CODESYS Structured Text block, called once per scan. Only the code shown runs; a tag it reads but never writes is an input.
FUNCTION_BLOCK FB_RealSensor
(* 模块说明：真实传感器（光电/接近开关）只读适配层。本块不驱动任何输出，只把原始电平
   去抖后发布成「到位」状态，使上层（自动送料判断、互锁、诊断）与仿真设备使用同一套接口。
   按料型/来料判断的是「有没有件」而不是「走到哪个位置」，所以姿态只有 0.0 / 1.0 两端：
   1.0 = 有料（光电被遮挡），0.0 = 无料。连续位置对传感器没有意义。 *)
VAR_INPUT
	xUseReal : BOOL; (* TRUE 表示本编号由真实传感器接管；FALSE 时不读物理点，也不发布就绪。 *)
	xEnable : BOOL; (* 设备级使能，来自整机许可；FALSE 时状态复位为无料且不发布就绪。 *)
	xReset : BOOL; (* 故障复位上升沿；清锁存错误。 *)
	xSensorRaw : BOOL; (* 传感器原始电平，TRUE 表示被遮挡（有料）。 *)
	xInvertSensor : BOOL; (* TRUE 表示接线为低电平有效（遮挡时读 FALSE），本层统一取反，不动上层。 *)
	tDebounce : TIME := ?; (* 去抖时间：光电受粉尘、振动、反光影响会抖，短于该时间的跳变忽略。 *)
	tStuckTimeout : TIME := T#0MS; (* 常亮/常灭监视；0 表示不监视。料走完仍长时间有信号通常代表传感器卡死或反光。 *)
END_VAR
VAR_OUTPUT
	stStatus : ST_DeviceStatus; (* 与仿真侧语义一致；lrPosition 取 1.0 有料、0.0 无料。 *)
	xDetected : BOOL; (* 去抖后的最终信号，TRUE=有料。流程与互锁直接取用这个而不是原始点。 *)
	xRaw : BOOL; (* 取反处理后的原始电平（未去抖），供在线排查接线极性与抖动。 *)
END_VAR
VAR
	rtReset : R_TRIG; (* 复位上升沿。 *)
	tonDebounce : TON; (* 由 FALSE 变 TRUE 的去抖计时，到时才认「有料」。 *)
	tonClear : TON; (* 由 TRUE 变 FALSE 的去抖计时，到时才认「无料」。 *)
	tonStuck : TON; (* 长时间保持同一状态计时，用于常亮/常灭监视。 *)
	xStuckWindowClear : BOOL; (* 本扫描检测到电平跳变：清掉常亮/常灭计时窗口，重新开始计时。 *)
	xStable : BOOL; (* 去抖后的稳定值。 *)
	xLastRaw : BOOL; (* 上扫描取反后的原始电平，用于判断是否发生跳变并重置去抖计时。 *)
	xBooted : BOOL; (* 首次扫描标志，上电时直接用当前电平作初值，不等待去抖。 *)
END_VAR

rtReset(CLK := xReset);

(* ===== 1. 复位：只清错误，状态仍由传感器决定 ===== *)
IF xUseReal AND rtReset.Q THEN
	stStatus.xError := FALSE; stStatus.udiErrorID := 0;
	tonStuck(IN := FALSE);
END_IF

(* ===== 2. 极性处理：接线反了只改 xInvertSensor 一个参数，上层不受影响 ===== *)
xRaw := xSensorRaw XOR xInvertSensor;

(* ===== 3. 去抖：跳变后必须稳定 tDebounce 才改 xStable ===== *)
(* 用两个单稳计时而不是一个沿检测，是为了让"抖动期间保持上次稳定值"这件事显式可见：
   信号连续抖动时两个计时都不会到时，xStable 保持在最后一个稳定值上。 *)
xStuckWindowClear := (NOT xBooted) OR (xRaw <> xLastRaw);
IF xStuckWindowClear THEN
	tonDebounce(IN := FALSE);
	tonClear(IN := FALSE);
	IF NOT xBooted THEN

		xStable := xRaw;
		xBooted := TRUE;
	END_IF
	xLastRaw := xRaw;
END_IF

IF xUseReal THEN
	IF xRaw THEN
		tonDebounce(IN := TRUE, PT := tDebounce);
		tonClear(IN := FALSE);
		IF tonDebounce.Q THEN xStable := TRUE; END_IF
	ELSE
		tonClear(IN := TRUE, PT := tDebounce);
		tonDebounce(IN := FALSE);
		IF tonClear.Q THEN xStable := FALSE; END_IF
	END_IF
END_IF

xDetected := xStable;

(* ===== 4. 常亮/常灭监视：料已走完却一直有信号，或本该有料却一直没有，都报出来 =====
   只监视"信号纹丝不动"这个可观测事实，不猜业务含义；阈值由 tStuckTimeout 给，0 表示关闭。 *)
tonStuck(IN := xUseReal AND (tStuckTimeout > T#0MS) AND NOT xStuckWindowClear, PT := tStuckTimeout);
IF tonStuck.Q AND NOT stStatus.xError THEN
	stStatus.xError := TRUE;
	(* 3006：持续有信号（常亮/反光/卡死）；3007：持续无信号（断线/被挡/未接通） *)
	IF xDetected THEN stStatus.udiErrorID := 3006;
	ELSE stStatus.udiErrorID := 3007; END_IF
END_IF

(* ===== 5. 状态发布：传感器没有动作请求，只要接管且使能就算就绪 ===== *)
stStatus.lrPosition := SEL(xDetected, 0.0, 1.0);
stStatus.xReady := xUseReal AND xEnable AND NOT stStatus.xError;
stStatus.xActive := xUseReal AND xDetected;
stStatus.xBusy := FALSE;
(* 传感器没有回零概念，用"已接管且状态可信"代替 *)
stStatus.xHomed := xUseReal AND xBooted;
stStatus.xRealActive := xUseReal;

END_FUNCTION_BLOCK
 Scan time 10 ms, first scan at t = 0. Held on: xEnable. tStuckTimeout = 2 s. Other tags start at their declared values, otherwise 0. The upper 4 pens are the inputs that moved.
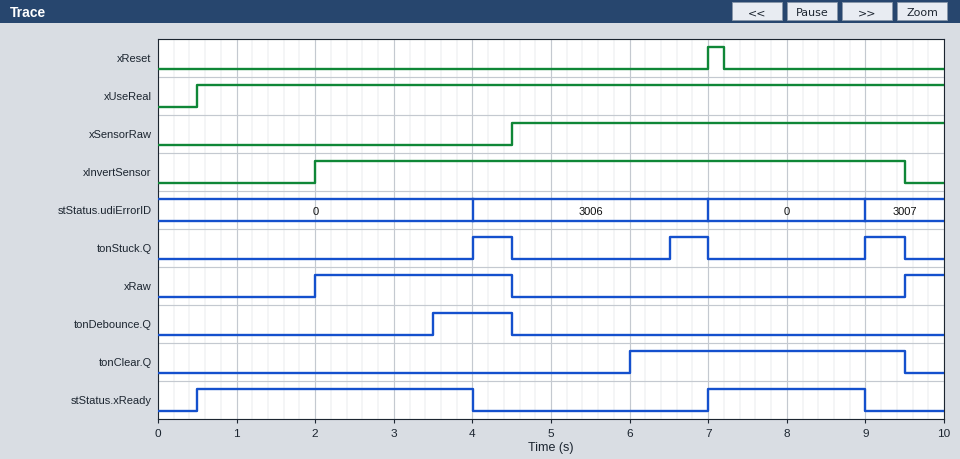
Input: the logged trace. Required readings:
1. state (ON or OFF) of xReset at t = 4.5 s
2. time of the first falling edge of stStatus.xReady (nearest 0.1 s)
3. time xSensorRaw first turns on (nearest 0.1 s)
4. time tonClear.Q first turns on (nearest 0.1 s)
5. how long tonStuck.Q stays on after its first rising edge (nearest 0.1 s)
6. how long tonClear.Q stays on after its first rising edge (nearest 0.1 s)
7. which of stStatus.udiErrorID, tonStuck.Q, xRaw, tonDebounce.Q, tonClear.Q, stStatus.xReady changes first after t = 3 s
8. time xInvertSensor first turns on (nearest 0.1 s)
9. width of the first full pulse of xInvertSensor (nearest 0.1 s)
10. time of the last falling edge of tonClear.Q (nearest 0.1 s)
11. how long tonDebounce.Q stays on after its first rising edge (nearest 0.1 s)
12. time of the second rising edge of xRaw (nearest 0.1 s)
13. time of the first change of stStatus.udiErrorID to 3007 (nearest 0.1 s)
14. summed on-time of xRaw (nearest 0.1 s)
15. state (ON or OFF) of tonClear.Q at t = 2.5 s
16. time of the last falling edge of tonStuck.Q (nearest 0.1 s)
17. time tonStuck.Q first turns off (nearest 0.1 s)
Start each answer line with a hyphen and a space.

- OFF
- 4.0 s
- 4.5 s
- 6.0 s
- 0.5 s
- 3.5 s
- tonDebounce.Q
- 2.0 s
- 7.5 s
- 9.5 s
- 1.0 s
- 9.5 s
- 9.0 s
- 3.0 s
- OFF
- 9.5 s
- 4.5 s
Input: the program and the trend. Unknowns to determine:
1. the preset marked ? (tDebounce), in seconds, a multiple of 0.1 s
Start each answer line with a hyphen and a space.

- 1.5 s
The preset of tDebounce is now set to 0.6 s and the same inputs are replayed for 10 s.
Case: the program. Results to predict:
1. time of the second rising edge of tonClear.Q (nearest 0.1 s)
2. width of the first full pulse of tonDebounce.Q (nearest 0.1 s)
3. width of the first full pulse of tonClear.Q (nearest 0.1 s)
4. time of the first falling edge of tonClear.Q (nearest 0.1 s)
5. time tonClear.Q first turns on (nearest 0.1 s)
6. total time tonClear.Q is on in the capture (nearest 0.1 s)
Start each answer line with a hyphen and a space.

- 5.1 s
- 1.9 s
- 0.9 s
- 2.0 s
- 1.1 s
- 5.3 s
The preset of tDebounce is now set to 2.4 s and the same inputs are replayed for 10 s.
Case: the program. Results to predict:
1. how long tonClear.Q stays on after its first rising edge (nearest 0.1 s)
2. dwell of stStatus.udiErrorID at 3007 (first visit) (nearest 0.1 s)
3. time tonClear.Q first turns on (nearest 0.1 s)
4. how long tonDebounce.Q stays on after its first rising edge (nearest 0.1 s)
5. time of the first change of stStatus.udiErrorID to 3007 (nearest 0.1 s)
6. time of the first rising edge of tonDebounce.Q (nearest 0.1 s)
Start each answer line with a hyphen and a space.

- 2.6 s
- 3.0 s
- 6.9 s
- 0.1 s
- 4.0 s
- 4.4 s
